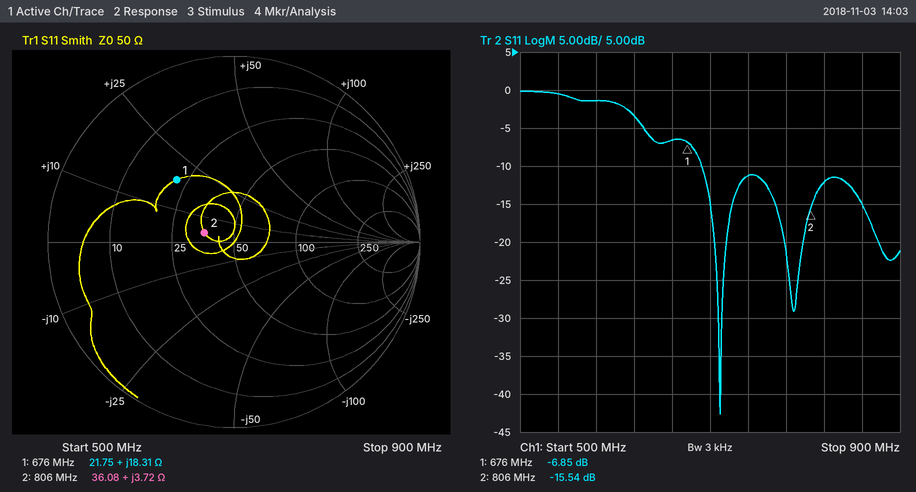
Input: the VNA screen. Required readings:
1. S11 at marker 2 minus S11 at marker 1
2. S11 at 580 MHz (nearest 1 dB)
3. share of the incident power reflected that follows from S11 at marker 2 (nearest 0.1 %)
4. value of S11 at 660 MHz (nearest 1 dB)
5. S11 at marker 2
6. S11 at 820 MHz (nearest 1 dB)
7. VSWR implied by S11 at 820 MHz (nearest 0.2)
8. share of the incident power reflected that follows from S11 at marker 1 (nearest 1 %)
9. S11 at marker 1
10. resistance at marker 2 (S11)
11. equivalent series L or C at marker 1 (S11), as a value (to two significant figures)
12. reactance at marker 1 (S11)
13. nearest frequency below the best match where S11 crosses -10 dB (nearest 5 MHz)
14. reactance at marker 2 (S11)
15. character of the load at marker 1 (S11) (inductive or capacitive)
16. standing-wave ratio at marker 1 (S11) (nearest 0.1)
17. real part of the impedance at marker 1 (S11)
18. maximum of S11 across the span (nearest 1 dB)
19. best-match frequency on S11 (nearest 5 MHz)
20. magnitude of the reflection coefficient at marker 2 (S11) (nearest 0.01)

-8.69 dB
-1 dB
2.8 %
-7 dB
-15.54 dB
-12 dB
1.6
21 %
-6.85 dB
36.08 Ω
4.3 nH
+18.31 Ω
690 MHz
+3.72 Ω
inductive
2.7
21.75 Ω
0 dB
710 MHz
0.17
